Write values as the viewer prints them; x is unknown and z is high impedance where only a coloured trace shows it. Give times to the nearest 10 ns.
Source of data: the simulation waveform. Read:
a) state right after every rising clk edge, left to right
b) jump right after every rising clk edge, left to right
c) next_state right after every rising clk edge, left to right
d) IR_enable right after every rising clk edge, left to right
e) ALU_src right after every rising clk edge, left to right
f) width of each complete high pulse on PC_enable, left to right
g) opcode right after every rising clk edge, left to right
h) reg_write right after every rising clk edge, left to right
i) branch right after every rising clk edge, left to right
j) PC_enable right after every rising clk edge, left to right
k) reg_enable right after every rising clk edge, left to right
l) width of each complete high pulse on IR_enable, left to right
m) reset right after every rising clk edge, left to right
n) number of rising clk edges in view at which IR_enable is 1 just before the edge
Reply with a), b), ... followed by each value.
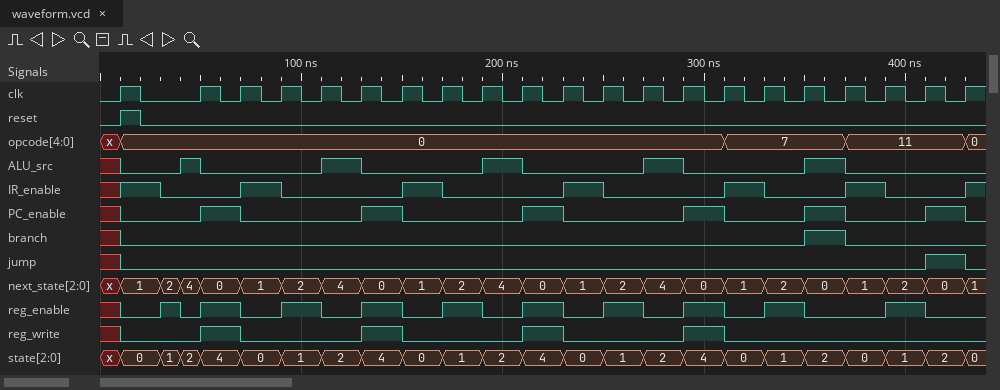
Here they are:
a) 0, 4, 0, 1, 2, 4, 0, 1, 2, 4, 0, 1, 2, 4, 0, 1, 2, 0, 1, 2, 0
b) 0 0 0 0 0 0 0 0 0 0 0 0 0 0 0 0 0 0 0 1 0
c) 1, 0, 1, 2, 4, 0, 1, 2, 4, 0, 1, 2, 4, 0, 1, 2, 0, 1, 2, 0, 1
d) 1 0 1 0 0 0 1 0 0 0 1 0 0 0 1 0 0 1 0 0 1
e) 0 0 0 0 1 0 0 0 1 0 0 0 1 0 0 0 1 0 0 0 0
f) 20 ns, 20 ns, 20 ns, 20 ns, 20 ns, 20 ns
g) 0, 0, 0, 0, 0, 0, 0, 0, 0, 0, 0, 0, 0, 0, 7, 7, 7, 11, 11, 11, 0
h) 0 1 0 0 0 1 0 0 0 1 0 0 0 1 0 0 0 0 0 0 0
i) 0 0 0 0 0 0 0 0 0 0 0 0 0 0 0 0 1 0 0 0 0
j) 0 1 0 0 0 1 0 0 0 1 0 0 0 1 0 0 1 0 0 1 0
k) 0 1 0 1 0 1 0 1 0 1 0 1 0 1 0 1 0 0 1 0 0
l) 20 ns, 20 ns, 20 ns, 20 ns, 20 ns
m) 1 0 0 0 0 0 0 0 0 0 0 0 0 0 0 0 0 0 0 0 0
n) 5
